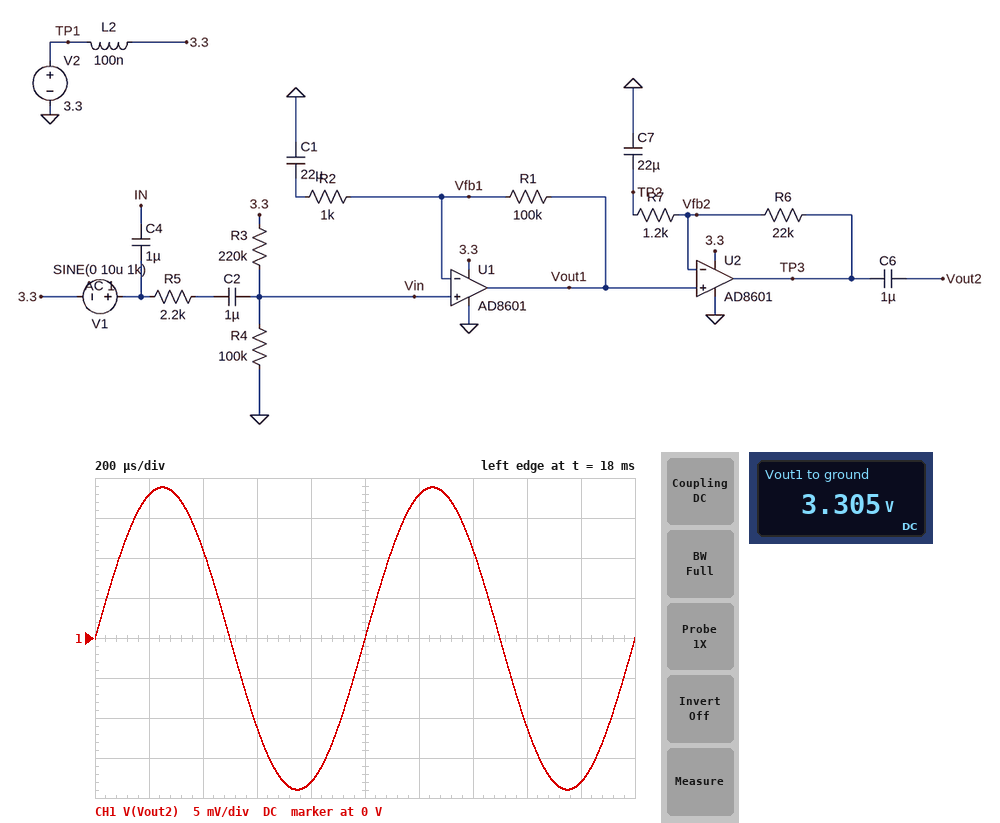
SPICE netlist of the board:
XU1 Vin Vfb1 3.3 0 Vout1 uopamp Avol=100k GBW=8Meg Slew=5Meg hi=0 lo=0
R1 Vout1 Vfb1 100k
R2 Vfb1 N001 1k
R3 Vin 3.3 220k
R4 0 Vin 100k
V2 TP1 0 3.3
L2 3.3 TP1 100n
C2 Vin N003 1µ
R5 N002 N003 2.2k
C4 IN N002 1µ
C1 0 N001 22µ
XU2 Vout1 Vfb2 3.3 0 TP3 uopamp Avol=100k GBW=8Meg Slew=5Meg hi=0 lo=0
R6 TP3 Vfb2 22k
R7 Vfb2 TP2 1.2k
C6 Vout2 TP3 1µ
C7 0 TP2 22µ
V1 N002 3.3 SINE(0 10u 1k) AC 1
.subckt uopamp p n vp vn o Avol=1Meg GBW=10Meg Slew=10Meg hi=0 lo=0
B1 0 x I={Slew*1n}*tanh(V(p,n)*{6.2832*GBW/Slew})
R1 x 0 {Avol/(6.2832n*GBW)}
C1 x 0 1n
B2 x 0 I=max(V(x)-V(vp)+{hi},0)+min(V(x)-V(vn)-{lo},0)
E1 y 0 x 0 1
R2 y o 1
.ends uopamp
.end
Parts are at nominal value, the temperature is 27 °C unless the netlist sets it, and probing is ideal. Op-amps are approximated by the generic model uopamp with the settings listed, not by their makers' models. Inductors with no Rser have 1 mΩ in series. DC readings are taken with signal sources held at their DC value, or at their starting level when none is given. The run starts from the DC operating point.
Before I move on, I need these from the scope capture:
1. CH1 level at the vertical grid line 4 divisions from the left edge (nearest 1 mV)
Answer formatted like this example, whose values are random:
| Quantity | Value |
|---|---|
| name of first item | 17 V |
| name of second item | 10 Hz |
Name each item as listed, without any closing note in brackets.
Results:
| Quantity | Value |
|---|---|
| CH1 level at the vertical grid line 4 divisions from the left edge | -18 mV |
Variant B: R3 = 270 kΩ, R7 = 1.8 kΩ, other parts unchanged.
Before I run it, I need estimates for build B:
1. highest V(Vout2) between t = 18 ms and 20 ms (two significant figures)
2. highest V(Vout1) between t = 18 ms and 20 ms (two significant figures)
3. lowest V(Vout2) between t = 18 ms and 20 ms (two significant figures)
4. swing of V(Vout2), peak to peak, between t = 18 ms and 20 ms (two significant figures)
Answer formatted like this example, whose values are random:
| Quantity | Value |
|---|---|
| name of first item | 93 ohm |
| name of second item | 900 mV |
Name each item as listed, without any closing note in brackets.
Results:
| Quantity | Value |
|---|---|
| highest V(Vout2) between t = 18 ms and 20 ms | 13 mV |
| highest V(Vout1) between t = 18 ms and 20 ms | 890 mV |
| lowest V(Vout2) between t = 18 ms and 20 ms | -13 mV |
| swing of V(Vout2), peak to peak, between t = 18 ms and 20 ms | 26 mV |
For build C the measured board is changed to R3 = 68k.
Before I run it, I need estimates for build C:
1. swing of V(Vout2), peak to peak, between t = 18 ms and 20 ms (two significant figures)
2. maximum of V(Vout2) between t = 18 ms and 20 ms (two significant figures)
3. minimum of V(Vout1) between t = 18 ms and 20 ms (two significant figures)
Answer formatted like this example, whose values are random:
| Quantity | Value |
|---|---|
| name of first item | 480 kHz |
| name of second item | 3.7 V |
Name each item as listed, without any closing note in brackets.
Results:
| Quantity | Value |
|---|---|
| swing of V(Vout2), peak to peak, between t = 18 ms and 20 ms | 37 mV |
| maximum of V(Vout2) between t = 18 ms and 20 ms | 18 mV |
| minimum of V(Vout1) between t = 18 ms and 20 ms | 2.0 V |
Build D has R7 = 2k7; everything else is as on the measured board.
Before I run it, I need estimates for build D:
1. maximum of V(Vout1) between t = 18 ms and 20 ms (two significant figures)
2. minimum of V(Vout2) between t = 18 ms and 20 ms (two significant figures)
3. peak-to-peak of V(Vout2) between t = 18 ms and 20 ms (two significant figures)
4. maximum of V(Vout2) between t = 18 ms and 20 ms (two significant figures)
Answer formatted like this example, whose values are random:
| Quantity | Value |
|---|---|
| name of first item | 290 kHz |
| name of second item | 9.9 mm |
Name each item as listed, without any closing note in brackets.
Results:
| Quantity | Value |
|---|---|
| maximum of V(Vout1) between t = 18 ms and 20 ms | 1.0 V |
| minimum of V(Vout2) between t = 18 ms and 20 ms | -9.0 mV |
| peak-to-peak of V(Vout2) between t = 18 ms and 20 ms | 18 mV |
| maximum of V(Vout2) between t = 18 ms and 20 ms | 8.9 mV |
